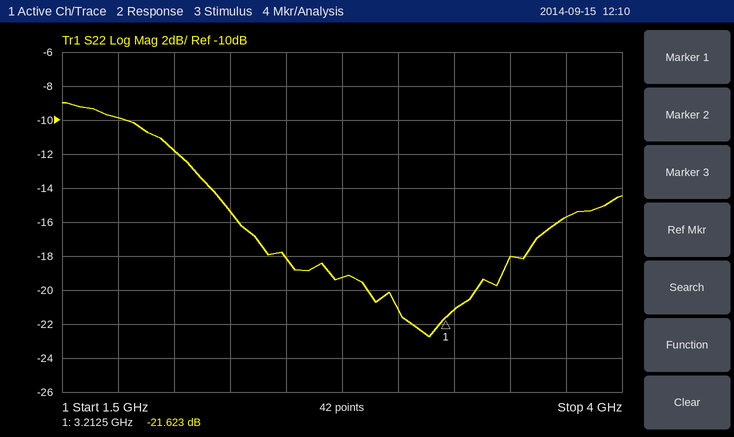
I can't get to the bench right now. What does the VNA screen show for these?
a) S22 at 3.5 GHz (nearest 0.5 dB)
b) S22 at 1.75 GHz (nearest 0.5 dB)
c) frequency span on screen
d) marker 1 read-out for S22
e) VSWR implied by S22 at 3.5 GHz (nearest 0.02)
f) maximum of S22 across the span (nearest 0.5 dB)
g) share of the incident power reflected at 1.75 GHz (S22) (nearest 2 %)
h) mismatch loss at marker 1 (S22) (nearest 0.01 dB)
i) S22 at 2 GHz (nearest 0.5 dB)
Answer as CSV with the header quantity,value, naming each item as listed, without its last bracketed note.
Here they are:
quantity,value
S22 at 3.5 GHz,-18.0 dB
S22 at 1.75 GHz,-10.0 dB
frequency span on screen,2.5 GHz
marker 1 read-out for S22,-21.623 dB
VSWR implied by S22 at 3.5 GHz,1.28
maximum of S22 across the span,-9.0 dB
share of the incident power reflected at 1.75 GHz (S22),10 %
mismatch loss at marker 1 (S22),0.03 dB
S22 at 2 GHz,-12.0 dB
